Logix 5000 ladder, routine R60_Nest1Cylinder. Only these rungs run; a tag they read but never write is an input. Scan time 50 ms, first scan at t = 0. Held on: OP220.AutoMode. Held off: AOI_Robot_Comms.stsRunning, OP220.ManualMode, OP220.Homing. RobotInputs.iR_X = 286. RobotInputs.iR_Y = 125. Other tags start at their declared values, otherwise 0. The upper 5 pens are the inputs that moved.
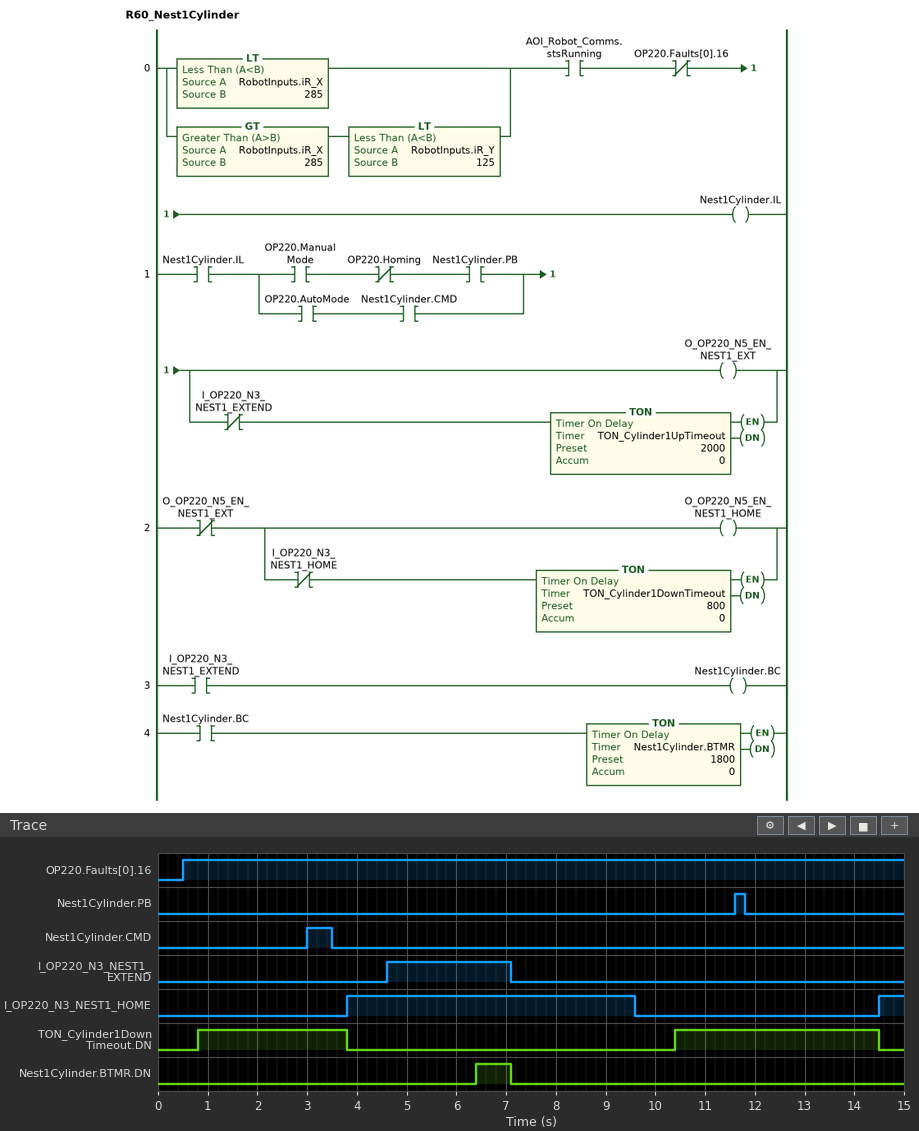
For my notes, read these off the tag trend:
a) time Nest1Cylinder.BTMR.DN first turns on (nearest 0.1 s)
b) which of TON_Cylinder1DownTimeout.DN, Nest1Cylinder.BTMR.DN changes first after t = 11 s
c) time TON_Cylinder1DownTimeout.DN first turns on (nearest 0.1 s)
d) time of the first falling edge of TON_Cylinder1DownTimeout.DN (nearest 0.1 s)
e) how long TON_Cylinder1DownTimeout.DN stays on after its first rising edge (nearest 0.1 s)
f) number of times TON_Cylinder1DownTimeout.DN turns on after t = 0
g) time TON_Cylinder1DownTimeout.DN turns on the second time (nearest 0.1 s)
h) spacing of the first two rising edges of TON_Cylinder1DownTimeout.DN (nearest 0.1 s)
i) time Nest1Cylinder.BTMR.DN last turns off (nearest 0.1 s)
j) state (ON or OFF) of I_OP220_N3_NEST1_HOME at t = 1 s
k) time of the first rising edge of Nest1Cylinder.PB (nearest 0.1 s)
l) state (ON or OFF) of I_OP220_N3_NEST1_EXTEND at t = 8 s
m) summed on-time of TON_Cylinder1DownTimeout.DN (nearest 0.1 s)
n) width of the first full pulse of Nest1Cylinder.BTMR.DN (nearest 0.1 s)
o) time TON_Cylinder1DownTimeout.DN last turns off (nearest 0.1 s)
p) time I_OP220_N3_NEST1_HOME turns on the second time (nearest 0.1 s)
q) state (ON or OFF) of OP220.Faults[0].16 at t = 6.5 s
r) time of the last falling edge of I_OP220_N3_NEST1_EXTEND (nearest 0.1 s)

6.4 s
TON_Cylinder1DownTimeout.DN
0.8 s
3.8 s
3.0 s
2
10.4 s
9.6 s
7.1 s
OFF
11.6 s
OFF
7.1 s
0.7 s
14.5 s
14.5 s
ON
7.1 s
